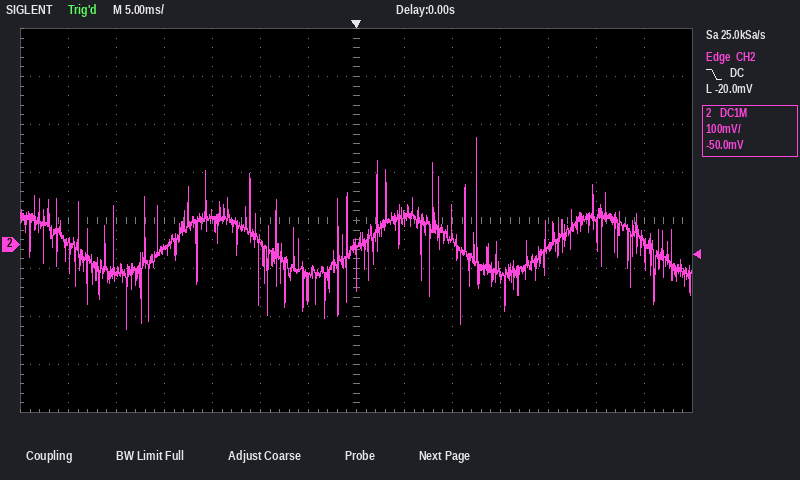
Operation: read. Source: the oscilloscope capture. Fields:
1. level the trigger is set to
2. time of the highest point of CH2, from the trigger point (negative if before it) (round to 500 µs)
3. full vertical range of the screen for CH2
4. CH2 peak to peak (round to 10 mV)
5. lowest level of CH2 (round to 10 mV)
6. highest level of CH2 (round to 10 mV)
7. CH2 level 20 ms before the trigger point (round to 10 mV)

-20.0 mV
+12.5 ms
800 mV
400 mV
-180 mV
220 mV
-10 mV
